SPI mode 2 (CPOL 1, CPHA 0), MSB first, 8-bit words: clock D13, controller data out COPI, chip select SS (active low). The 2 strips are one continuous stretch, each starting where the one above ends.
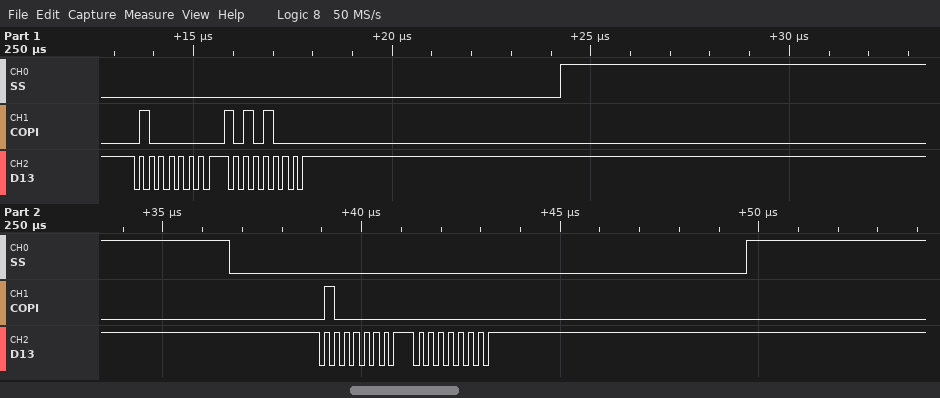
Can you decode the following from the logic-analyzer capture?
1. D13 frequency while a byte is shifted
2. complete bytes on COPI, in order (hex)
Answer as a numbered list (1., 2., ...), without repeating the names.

1. 4 MHz
2. 40 A8 40 00
